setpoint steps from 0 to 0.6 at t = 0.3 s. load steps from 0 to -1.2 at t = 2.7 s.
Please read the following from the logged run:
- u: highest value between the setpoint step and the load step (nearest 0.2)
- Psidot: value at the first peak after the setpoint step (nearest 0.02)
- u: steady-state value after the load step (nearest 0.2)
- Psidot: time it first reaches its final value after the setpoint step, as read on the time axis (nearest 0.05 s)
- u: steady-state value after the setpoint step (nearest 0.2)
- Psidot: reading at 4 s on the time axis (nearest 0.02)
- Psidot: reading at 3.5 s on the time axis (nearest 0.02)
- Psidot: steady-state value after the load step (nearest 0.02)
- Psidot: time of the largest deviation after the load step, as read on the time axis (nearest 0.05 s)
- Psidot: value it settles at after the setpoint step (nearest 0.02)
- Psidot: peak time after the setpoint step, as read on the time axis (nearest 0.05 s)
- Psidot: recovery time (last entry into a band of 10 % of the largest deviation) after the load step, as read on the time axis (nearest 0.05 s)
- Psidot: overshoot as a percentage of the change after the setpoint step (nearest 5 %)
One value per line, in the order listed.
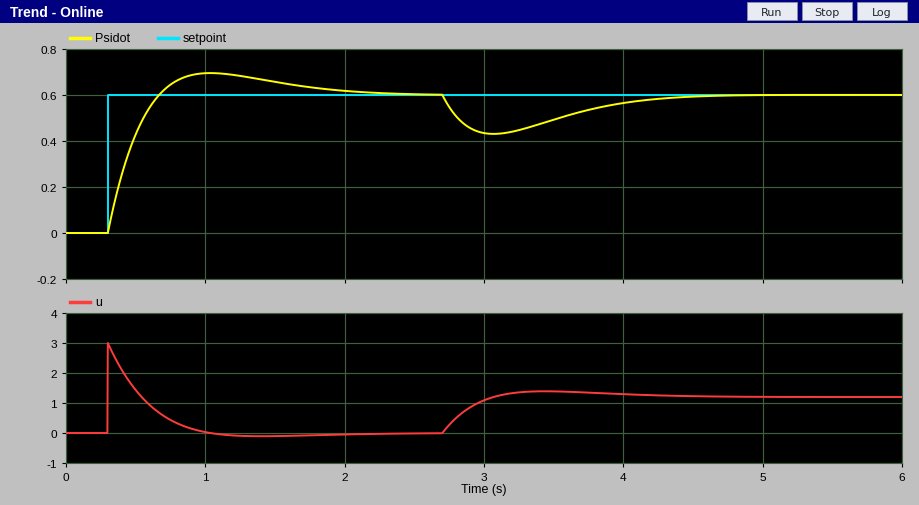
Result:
3.0
0.70
1.2
0.65 s
0.0
0.56
0.50
0.60
3.05 s
0.60
1.05 s
4.25 s
15 %
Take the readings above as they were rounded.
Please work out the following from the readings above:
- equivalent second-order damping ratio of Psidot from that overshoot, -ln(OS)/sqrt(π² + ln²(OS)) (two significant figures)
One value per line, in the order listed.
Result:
0.52
